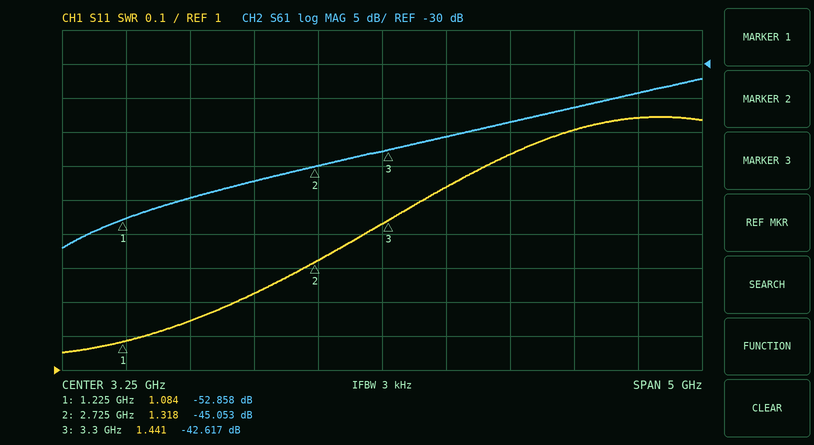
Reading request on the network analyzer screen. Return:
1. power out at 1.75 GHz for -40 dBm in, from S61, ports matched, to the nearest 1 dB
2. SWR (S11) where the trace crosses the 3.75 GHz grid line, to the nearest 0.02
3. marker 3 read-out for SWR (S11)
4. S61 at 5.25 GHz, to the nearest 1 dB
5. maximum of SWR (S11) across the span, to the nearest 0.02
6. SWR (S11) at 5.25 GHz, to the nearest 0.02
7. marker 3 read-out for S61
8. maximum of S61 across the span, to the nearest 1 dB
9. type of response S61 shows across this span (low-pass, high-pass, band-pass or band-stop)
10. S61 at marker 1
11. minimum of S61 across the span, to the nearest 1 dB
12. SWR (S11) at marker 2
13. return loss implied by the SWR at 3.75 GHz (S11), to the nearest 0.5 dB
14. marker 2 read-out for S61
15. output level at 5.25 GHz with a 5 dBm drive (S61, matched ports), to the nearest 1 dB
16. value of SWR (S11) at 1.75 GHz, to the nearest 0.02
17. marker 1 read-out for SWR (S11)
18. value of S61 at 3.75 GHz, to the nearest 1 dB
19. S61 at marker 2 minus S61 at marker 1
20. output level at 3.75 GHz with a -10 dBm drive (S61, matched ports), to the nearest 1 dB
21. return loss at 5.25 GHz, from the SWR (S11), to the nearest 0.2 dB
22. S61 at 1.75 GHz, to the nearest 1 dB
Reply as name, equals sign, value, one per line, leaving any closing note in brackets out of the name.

power out at 1.75 GHz for -40 dBm in, from S61, ports matched, to the nearest 1 dB = -90 dBm
SWR (S11) where the trace crosses the 3.75 GHz grid line, to the nearest 0.02 = 1.54
marker 3 read-out for SWR = 1.441
S61 at 5.25 GHz, to the nearest 1 dB = -34 dB
maximum of SWR (S11) across the span, to the nearest 0.02 = 1.74
SWR (S11) at 5.25 GHz, to the nearest 0.02 = 1.74
marker 3 read-out for S61 = -42.617 dB
maximum of S61 across the span, to the nearest 1 dB = -32 dB
type of response S61 shows across this span = high-pass
S61 at marker 1 = -52.858 dB
minimum of S61 across the span, to the nearest 1 dB = -57 dB
SWR (S11) at marker 2 = 1.318
return loss implied by the SWR at 3.75 GHz (S11), to the nearest 0.5 dB = 13.5 dB
marker 2 read-out for S61 = -45.053 dB
output level at 5.25 GHz with a 5 dBm drive (S61, matched ports), to the nearest 1 dB = -29 dBm
value of SWR (S11) at 1.75 GHz, to the nearest 0.02 = 1.14
marker 1 read-out for SWR = 1.084
value of S61 at 3.75 GHz, to the nearest 1 dB = -41 dB
S61 at marker 2 minus S61 at marker 1 = 7.805 dB
output level at 3.75 GHz with a -10 dBm drive (S61, matched ports), to the nearest 1 dB = -51 dBm
return loss at 5.25 GHz, from the SWR (S11), to the nearest 0.2 dB = 11.4 dB
S61 at 1.75 GHz, to the nearest 1 dB = -50 dB
